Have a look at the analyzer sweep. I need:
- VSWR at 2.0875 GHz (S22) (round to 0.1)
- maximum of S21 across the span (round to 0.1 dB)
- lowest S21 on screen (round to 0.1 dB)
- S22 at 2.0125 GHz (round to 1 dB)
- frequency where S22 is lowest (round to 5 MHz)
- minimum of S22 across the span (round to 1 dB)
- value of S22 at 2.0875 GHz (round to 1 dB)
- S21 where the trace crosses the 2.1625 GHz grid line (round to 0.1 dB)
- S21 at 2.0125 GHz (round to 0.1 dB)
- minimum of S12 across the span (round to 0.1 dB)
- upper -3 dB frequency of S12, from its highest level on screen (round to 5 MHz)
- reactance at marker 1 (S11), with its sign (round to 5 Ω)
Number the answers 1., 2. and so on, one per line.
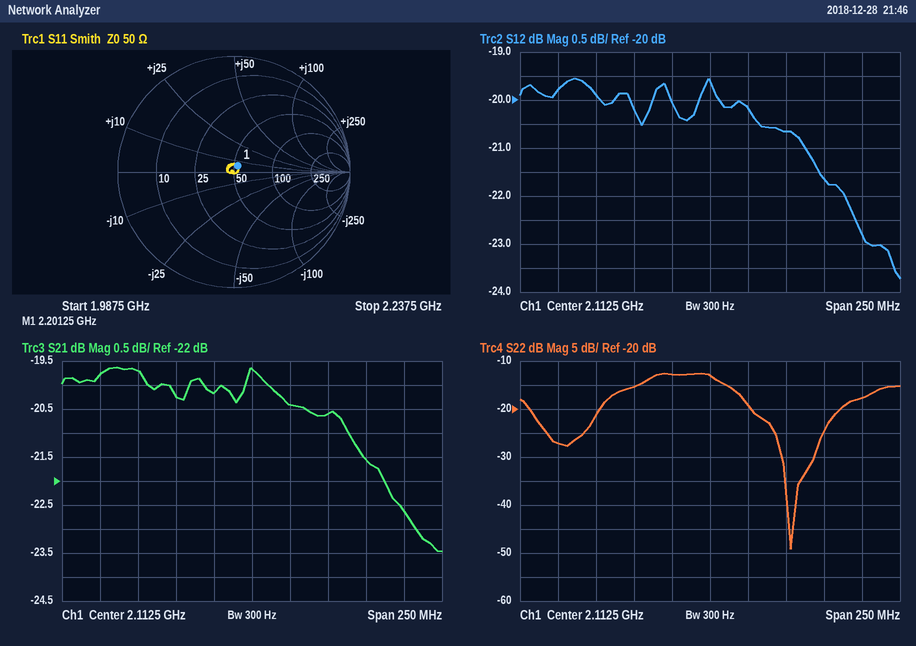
1. 1.6
2. -19.6 dB
3. -23.5 dB
4. -27 dB
5. 2.165 GHz
6. -49 dB
7. -13 dB
8. -20.6 dB
9. -19.8 dB
10. -23.7 dB
11. 2.210 GHz
12. +5 Ω
